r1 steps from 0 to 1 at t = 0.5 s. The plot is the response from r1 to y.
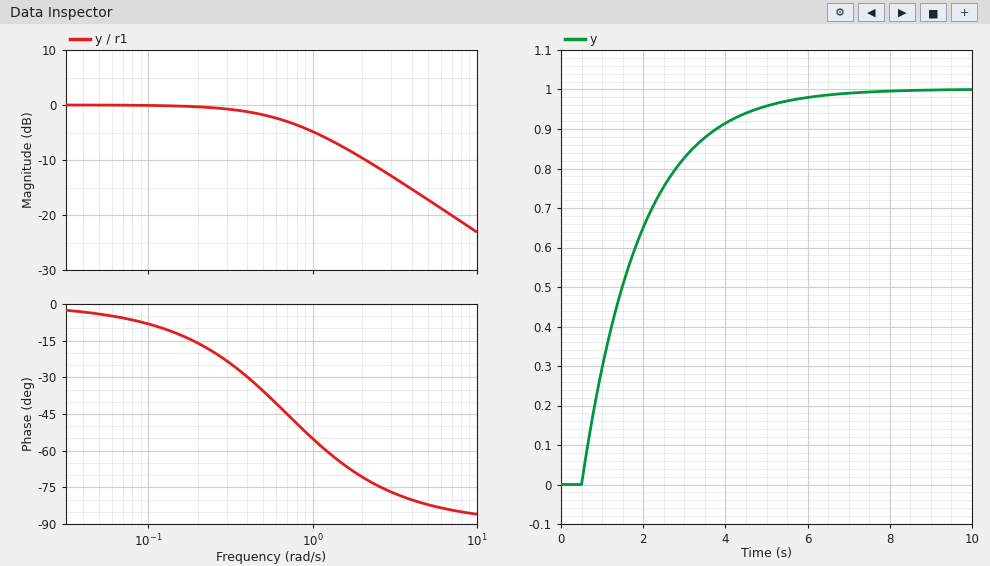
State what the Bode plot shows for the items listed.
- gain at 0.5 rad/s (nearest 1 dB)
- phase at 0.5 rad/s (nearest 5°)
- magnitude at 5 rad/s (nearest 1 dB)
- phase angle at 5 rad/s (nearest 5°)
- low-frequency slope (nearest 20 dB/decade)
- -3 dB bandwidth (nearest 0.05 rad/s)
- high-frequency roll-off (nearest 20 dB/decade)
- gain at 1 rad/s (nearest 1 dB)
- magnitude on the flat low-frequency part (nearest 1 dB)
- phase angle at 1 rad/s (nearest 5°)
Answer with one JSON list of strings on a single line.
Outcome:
["-2 dB", "-35°", "-17 dB", "-80°", "0 dB/decade", "0.70 rad/s", "-20 dB/decade", "-5 dB", "0 dB", "-55°"]
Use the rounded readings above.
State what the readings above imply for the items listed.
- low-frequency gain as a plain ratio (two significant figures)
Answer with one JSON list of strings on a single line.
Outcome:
["1.0"]
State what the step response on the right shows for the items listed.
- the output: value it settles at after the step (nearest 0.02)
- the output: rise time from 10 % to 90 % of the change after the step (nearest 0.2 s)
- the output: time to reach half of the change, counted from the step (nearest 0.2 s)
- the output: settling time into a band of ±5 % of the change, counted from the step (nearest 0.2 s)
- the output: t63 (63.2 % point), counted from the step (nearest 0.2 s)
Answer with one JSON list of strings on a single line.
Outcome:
["1.00", "3.2 s", "1.0 s", "4.2 s", "1.4 s"]
